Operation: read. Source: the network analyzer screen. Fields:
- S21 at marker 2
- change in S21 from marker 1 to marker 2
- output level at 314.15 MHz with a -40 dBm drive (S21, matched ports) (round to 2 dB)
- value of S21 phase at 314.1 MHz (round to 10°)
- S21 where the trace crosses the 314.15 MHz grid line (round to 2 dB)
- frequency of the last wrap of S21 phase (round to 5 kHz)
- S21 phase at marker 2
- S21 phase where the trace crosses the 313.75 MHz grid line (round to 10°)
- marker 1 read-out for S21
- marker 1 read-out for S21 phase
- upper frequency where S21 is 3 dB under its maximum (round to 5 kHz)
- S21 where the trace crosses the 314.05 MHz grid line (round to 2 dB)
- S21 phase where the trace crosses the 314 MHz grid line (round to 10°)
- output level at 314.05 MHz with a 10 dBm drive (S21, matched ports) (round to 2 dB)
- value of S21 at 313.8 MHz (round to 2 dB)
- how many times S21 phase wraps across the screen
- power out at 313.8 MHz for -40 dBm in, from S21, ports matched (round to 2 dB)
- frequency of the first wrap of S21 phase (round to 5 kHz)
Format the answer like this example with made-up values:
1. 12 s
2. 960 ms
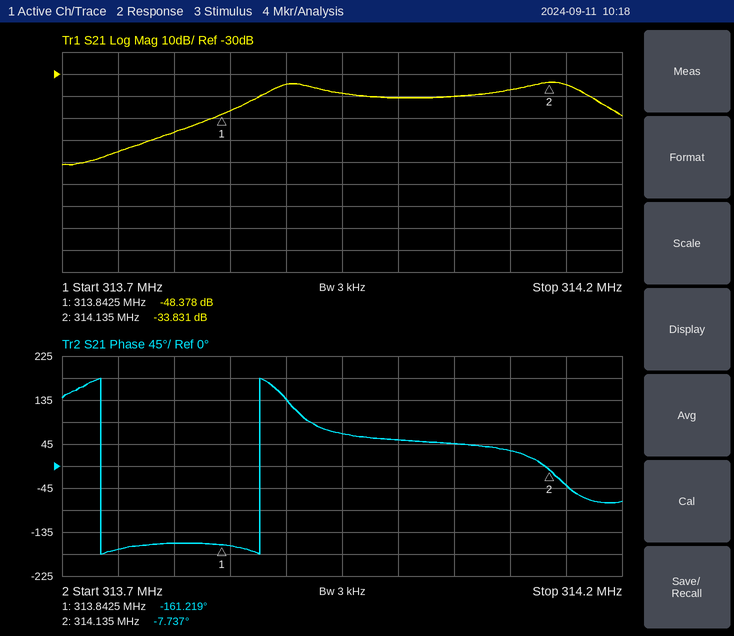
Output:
1. -33.831 dB
2. 14.547 dB
3. -74 dBm
4. 30°
5. -34 dB
6. 313.875 MHz
7. -7.737°
8. -170°
9. -48.378 dB
10. -161.219°
11. 314.160 MHz
12. -40 dB
13. 50°
14. -30 dBm
15. -56 dB
16. 2
17. -96 dBm
18. 313.735 MHz
